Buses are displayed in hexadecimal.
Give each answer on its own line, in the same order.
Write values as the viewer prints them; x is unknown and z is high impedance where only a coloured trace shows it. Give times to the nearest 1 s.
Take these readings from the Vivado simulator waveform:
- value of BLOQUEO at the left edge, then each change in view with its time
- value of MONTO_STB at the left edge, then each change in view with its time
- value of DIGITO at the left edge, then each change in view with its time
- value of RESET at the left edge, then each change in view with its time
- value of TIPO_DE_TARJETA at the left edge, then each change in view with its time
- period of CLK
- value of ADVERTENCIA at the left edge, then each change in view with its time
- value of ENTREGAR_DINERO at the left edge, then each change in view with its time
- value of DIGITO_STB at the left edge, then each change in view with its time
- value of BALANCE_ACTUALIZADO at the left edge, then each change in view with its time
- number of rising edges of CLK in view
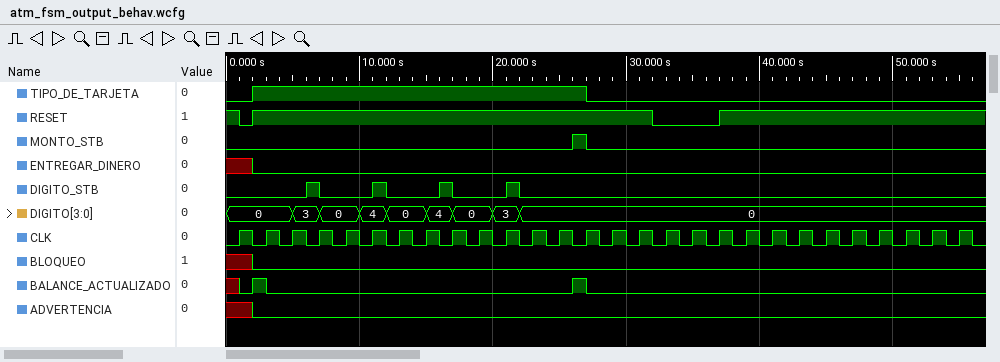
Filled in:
x, 0 at 2 s
0, 1 at 26 s, 0 at 27 s
0, 3 at 5 s, 0 at 7 s, 4 at 10 s, 0 at 12 s, 4 at 15 s, 0 at 17 s, 3 at 20 s, 0 at 22 s
1, 0 at 1 s, 1 at 2 s, 0 at 32 s, 1 at 37 s
0, 1 at 2 s, 0 at 27 s
2 s
x, 0 at 2 s
x, 0 at 2 s
0, 1 at 6 s, 0 at 7 s, 1 at 11 s, 0 at 12 s, 1 at 16 s, 0 at 17 s, 1 at 21 s, 0 at 22 s
x, 0 at 1 s, 1 at 2 s, 0 at 3 s, 1 at 26 s, 0 at 27 s
28
